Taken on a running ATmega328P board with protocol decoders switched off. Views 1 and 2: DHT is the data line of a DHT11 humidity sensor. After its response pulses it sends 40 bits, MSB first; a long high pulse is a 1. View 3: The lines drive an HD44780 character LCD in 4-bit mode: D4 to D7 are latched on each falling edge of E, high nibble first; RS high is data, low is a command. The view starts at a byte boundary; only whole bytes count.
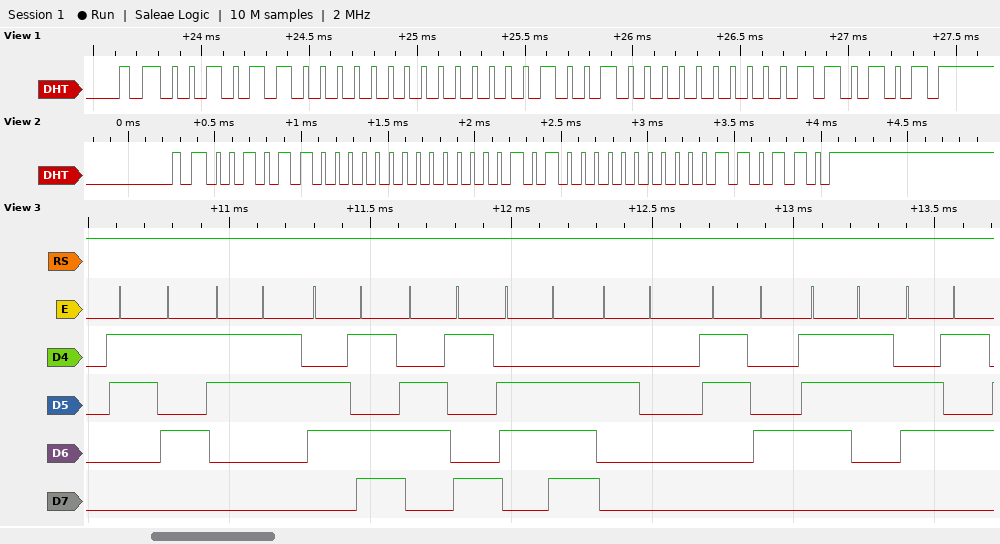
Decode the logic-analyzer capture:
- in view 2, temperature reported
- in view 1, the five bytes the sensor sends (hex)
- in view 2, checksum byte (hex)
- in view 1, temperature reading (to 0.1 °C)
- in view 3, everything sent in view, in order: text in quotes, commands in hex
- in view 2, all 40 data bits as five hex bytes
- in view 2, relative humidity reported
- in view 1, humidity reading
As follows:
10.0 °C
2C 00 09 00 35
0x36
9.0 °C
"53min 4se"
2C 00 0A 00 36
44 %
44 %
